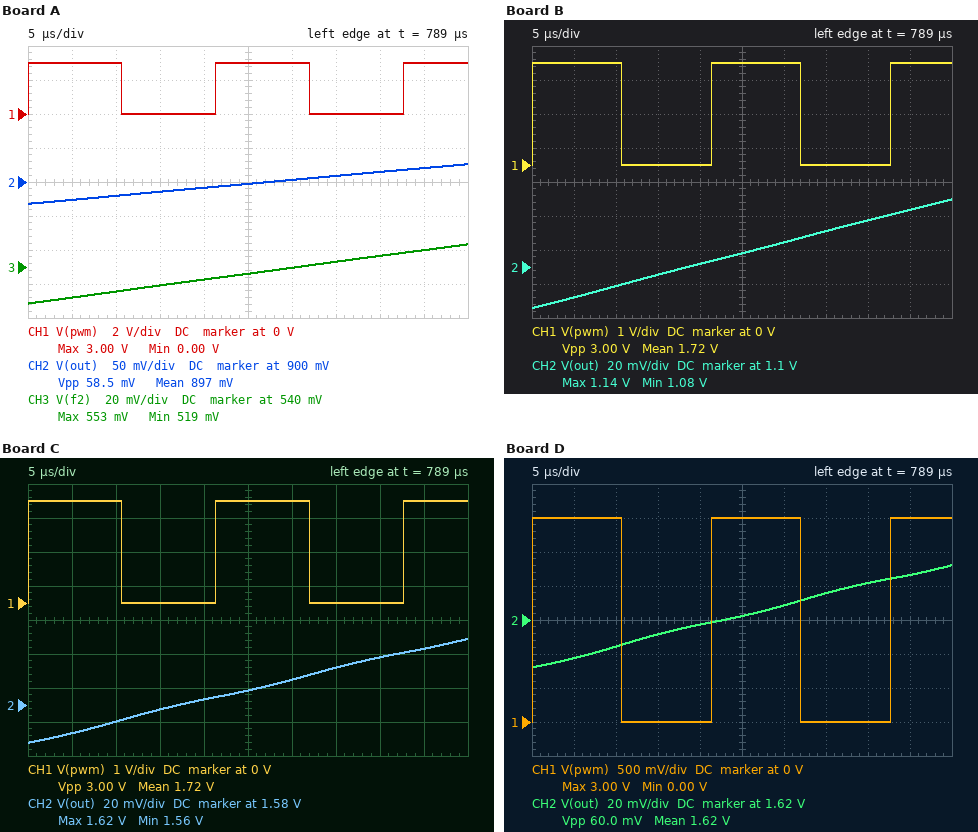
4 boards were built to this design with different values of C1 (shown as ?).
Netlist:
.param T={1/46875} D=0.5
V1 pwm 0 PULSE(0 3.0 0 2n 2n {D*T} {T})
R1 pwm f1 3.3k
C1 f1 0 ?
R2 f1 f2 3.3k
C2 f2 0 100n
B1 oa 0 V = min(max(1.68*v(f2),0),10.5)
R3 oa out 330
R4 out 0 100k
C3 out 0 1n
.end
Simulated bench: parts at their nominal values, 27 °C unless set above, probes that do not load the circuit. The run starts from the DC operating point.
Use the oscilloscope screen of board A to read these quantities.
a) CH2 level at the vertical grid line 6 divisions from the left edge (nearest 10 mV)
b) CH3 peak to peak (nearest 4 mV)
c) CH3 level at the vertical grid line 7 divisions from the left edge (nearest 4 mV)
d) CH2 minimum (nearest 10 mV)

900 mV
36 mV
544 mV
870 mV
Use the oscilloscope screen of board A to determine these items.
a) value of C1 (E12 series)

270 nF
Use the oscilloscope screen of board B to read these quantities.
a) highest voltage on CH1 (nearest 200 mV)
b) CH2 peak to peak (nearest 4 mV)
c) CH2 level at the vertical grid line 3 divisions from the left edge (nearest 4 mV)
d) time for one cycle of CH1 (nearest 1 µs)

3.0 V
64 mV
1.096 V
21 µs
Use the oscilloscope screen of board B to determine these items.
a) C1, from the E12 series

180 nF
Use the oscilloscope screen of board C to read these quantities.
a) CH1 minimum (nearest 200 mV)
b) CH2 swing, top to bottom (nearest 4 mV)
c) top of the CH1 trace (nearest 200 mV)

0 V
60 mV
3.0 V
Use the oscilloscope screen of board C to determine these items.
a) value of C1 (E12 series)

47 nF
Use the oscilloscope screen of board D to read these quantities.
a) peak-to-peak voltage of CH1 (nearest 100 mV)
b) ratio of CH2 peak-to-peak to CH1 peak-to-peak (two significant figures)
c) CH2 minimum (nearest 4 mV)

3.0 V
0.020
1.592 V
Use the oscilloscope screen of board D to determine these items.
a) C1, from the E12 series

39 nF
